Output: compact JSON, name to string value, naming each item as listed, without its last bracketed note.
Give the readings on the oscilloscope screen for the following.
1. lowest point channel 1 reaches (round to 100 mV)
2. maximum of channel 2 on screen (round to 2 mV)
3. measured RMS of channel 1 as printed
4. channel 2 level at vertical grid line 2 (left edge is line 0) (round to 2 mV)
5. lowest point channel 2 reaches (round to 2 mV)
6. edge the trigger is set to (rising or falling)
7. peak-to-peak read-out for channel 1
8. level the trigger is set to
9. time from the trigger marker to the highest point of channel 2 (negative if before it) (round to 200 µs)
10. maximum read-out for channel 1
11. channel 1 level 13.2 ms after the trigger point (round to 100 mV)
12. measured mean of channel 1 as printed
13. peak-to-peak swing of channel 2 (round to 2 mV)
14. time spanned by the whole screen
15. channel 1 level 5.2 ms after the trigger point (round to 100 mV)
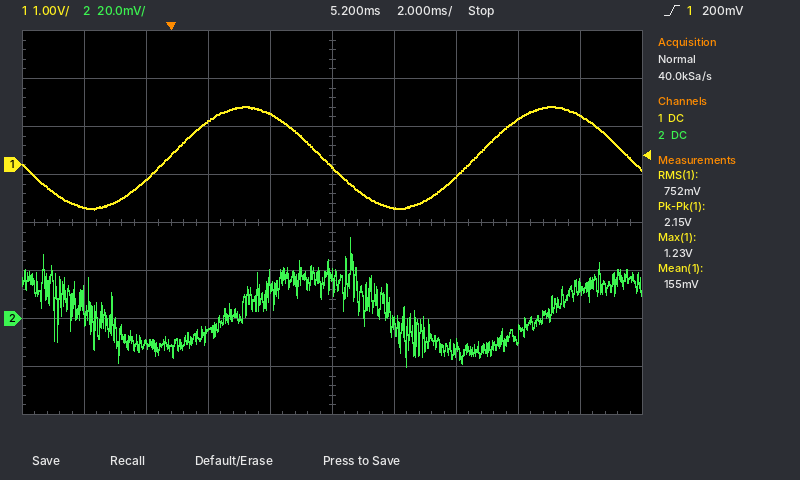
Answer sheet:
{"lowest point channel 1 reaches": "-900 mV", "maximum of channel 2 on screen": "34 mV", "measured RMS of channel 1 as printed": "752 mV", "channel 2 level at vertical grid line 2 (left edge is line 0)": "-10 mV", "lowest point channel 2 reaches": "-20 mV", "edge the trigger is set to": "rising", "peak-to-peak read-out for channel 1": "2.15 V", "level the trigger is set to": "200 mV", "time from the trigger marker to the highest point of channel 2 (negative if before it)": "+5.8 ms", "maximum read-out for channel 1": "1.23 V", "channel 1 level 13.2 ms after the trigger point": "1.0 V", "measured mean of channel 1 as printed": "155 mV", "peak-to-peak swing of channel 2": "54 mV", "time spanned by the whole screen": "20 ms", "channel 1 level 5.2 ms after the trigger point": "0.0 V"}
